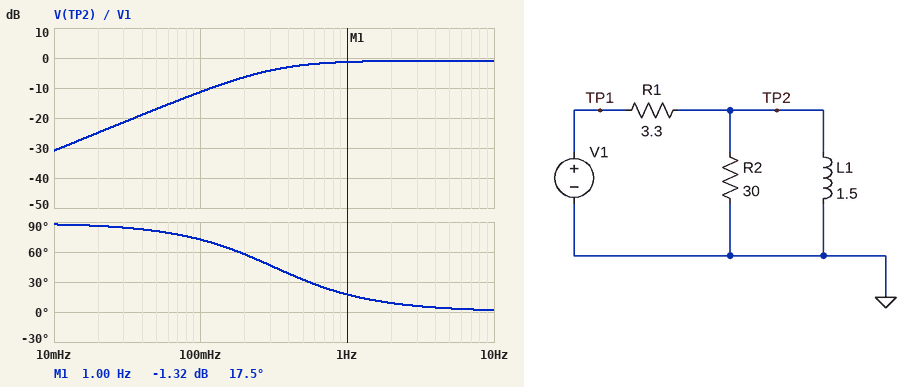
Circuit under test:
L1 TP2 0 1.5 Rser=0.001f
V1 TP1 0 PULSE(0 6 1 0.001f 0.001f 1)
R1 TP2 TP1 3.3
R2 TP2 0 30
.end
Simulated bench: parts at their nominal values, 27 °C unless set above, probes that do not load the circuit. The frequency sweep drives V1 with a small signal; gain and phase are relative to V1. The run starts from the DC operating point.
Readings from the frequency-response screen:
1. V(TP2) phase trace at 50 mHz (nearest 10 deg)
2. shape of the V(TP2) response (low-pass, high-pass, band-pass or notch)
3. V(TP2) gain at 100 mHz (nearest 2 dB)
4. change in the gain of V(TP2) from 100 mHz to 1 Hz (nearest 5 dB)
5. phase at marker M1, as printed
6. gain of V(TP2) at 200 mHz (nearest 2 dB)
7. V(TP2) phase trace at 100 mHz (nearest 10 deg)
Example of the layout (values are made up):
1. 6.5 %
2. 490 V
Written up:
1. 80 deg
2. high-pass
3. -12 dB
4. 10 dB
5. 17.5 deg
6. -6 dB
7. 70 deg
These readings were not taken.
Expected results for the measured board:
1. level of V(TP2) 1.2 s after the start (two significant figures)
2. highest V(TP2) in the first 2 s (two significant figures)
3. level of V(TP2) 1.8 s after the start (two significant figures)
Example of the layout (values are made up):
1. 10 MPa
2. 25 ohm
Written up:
1. 3.6 V
2. 5.4 V
3. 1.1 V
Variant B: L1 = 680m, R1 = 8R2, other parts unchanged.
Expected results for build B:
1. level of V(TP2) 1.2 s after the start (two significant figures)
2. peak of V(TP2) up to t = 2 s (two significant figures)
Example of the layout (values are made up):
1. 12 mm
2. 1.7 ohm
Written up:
1. 710 mV
2. 4.7 V
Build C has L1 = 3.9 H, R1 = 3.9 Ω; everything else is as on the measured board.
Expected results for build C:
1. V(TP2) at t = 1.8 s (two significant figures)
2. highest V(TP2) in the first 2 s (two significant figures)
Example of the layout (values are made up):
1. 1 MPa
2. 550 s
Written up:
1. 2.6 V
2. 5.3 V
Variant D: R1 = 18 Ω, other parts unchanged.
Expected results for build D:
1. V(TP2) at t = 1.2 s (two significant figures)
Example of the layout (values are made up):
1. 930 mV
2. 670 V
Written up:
1. 840 mV
